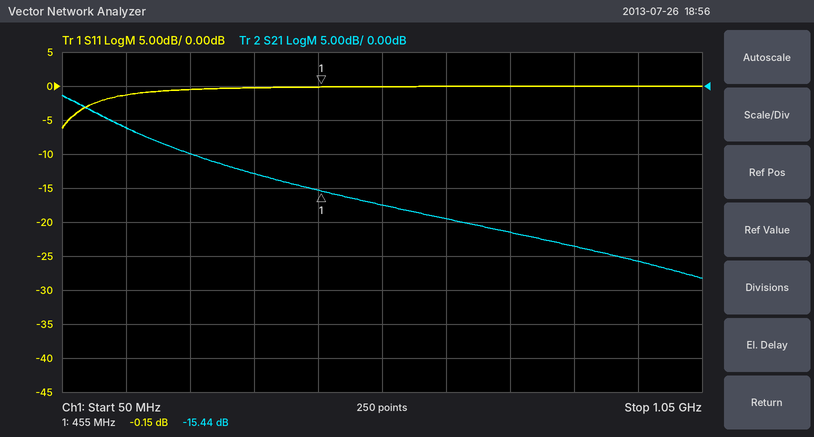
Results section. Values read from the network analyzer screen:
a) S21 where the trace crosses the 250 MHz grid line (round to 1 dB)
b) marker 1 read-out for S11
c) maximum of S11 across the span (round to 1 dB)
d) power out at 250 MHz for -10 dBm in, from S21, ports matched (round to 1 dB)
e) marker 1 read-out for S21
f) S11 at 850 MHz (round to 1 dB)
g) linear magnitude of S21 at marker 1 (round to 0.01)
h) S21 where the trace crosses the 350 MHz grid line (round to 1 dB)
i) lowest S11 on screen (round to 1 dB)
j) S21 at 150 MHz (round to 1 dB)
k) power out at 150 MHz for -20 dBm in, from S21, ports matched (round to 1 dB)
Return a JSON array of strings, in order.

["-10 dB", "-0.15 dB", "0 dB", "-20 dBm", "-15.44 dB", "0 dB", "0.17", "-13 dB", "-6 dB", "-6 dB", "-26 dBm"]
